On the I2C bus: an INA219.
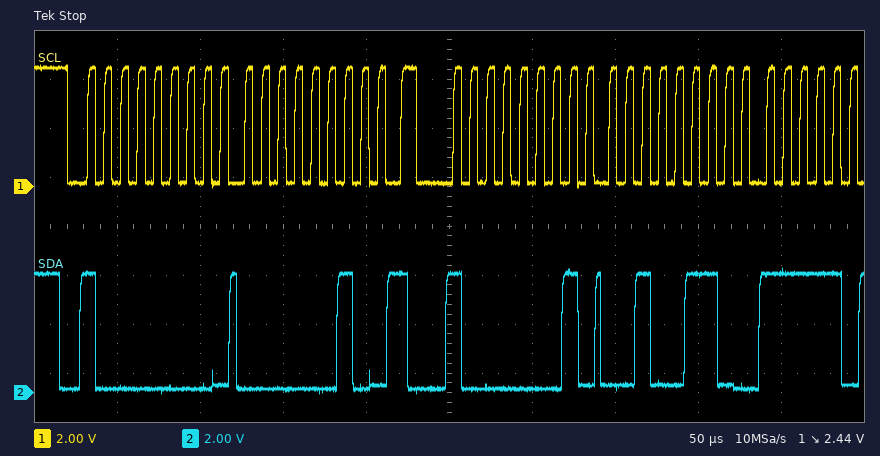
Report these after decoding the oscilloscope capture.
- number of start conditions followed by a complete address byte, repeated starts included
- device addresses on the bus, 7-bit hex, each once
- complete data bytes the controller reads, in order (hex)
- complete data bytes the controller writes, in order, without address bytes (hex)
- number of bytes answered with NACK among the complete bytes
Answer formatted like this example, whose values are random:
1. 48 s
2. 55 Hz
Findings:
1. 2
2. 0x40
3. 26
4. 02
5. 0
